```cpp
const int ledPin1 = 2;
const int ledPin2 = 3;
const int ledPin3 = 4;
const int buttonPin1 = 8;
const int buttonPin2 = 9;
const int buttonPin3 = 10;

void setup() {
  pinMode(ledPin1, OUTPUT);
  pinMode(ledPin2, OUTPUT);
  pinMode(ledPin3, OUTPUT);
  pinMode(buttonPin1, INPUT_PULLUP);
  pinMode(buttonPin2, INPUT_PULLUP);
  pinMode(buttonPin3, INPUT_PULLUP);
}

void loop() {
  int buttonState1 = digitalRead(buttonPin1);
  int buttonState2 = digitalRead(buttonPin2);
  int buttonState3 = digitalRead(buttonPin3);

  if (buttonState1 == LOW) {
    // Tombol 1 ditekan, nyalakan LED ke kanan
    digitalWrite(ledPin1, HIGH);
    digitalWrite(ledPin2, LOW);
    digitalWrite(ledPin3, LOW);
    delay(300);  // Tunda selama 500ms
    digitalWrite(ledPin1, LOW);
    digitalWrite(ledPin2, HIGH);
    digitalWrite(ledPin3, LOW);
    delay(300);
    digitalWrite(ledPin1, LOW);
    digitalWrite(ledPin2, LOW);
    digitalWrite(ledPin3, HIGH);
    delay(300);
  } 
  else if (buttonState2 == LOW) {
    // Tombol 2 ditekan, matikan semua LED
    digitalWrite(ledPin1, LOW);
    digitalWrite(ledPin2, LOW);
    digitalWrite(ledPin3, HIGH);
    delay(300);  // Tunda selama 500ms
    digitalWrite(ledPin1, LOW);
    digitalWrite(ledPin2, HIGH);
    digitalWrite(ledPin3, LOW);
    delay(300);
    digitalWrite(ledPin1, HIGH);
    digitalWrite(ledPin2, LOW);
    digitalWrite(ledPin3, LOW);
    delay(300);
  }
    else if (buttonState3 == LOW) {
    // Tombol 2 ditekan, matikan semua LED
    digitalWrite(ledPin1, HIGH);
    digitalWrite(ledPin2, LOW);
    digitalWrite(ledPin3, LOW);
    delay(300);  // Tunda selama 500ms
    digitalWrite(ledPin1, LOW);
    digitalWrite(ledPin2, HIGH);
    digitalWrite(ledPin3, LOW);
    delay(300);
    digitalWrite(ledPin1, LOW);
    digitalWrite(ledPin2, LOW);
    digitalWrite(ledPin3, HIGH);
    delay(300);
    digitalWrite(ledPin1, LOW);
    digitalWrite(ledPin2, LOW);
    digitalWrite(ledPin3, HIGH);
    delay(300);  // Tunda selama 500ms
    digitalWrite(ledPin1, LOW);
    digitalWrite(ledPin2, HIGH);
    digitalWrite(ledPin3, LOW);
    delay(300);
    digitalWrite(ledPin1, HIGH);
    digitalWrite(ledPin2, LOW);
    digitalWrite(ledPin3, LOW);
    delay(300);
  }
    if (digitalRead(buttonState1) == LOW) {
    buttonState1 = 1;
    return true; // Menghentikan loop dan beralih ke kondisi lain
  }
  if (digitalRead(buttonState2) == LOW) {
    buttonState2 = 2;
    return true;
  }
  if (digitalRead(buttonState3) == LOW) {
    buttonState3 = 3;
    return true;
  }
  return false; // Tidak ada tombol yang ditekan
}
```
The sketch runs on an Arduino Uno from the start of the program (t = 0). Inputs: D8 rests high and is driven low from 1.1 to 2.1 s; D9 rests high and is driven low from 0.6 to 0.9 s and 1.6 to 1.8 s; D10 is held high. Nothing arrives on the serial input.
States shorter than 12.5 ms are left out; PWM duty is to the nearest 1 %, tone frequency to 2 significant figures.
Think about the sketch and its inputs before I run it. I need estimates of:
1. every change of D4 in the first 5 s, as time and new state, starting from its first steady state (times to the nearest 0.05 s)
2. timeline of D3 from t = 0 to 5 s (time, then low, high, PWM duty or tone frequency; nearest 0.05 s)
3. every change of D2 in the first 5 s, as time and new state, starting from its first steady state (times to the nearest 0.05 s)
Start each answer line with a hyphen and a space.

- 0 s low; 0.6 s high; 0.9 s low; 2.1 s high
- 0 s low; 0.9 s high; 1.2 s low; 1.8 s high; 2.1 s low
- 0 s low; 1.2 s high; 1.8 s low
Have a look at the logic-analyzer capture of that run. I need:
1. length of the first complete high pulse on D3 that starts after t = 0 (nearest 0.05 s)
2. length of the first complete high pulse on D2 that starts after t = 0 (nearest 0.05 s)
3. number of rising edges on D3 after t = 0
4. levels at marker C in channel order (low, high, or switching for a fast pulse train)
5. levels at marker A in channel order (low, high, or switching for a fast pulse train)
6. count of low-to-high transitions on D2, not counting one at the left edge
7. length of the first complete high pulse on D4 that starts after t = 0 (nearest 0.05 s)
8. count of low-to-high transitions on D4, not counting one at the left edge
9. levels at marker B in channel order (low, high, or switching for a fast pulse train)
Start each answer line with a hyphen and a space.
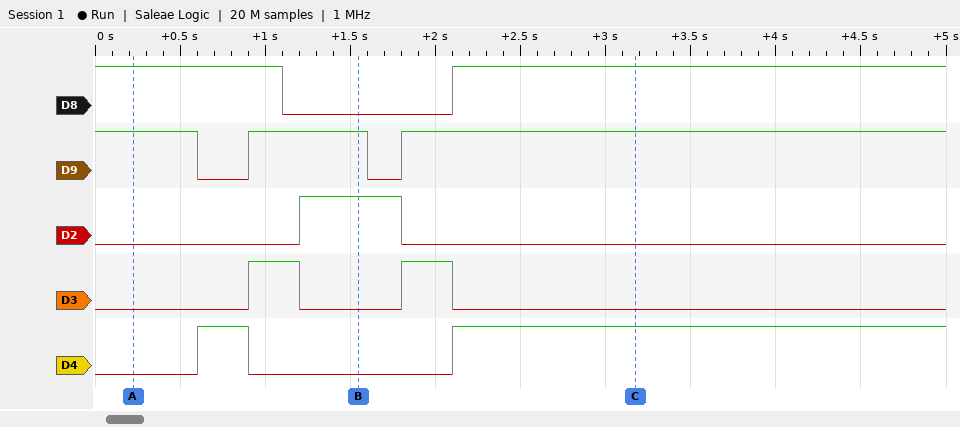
- 0.30 s
- 0.60 s
- 2
- D8 high, D9 high, D2 low, D3 low, D4 high
- D8 high, D9 high, D2 low, D3 low, D4 low
- 1
- 0.30 s
- 2
- D8 low, D9 high, D2 high, D3 low, D4 low
